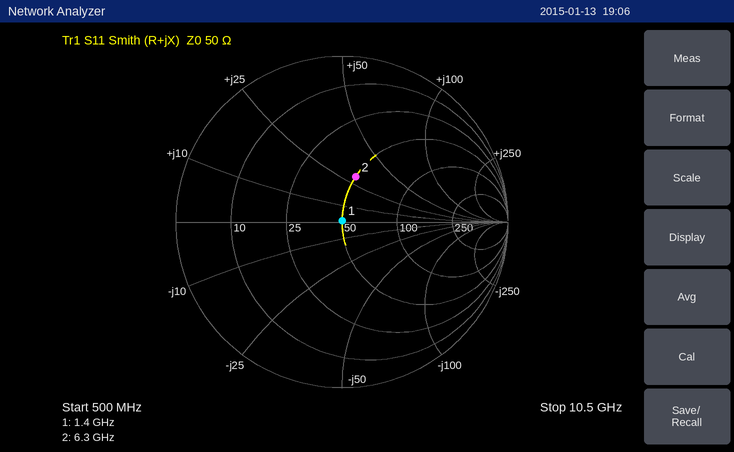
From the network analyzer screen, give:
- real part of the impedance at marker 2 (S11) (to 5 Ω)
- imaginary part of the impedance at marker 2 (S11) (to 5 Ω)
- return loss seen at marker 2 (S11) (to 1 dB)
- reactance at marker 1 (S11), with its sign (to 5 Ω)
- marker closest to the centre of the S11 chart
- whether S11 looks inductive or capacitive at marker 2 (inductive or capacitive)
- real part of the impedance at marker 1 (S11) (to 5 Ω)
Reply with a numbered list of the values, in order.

1. 50 Ω
2. +30 Ω
3. 11 dB
4. 0 Ω
5. marker 1
6. inductive
7. 50 Ω
